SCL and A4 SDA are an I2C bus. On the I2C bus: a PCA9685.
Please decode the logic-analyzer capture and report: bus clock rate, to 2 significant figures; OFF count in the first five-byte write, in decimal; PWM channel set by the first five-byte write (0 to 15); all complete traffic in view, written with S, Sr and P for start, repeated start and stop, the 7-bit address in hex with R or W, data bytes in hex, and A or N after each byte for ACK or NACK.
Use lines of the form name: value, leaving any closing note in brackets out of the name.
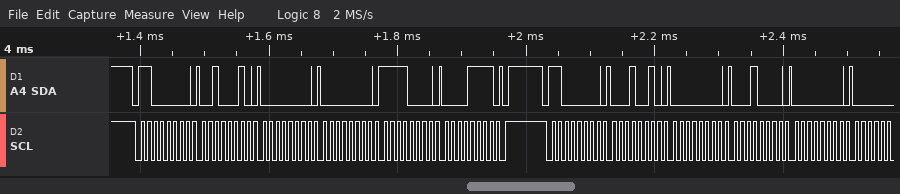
bus clock rate, to 2 significant figures: 100 kHz
OFF count in the first five-byte write, in decimal: 4080
PWM channel set by the first five-byte write: 7
all complete traffic in view, written with S, Sr and P for start, repeated start and stop, the 7-bit address in hex with R or W, data bytes in hex, and A or N after each byte for ACK or NACK: S 60W A 22 A 00 A 00 A F0 A 0F A P S 60W A 12 A 00 A 10 A 00 A
